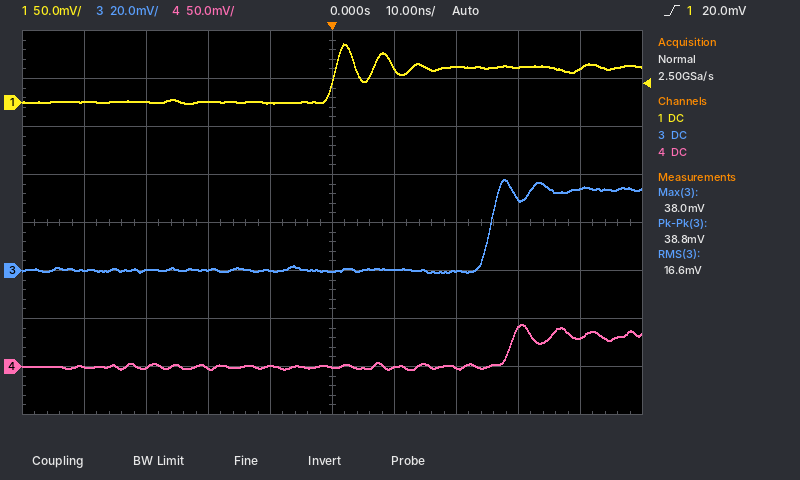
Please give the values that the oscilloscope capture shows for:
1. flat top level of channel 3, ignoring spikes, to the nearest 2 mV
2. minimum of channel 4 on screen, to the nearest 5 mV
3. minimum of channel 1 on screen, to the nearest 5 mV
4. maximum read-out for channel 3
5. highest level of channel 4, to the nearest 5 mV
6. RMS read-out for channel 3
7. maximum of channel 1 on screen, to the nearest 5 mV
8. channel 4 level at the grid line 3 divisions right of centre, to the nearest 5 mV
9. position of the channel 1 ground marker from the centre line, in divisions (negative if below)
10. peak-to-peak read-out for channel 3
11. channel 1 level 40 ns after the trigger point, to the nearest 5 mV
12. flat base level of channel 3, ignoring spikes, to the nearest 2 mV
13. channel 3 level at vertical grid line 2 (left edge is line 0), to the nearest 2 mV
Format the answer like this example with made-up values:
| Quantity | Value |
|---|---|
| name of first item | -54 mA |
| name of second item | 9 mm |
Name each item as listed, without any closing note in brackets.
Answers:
| Quantity | Value |
|---|---|
| flat top level of channel 3, ignoring spikes, to the nearest 2 mV | 34 mV |
| minimum of channel 4 on screen, to the nearest 5 mV | -5 mV |
| minimum of channel 1 on screen, to the nearest 5 mV | 0 mV |
| maximum read-out for channel 3 | 38.0 mV |
| highest level of channel 4, to the nearest 5 mV | 45 mV |
| RMS read-out for channel 3 | 16.6 mV |
| maximum of channel 1 on screen, to the nearest 5 mV | 60 mV |
| channel 4 level at the grid line 3 divisions right of centre, to the nearest 5 mV | 40 mV |
| position of the channel 1 ground marker from the centre line, in divisions | +2.5 div |
| peak-to-peak read-out for channel 3 | 38.8 mV |
| channel 1 level 40 ns after the trigger point, to the nearest 5 mV | 35 mV |
| flat base level of channel 3, ignoring spikes, to the nearest 2 mV | 0 mV |
| channel 3 level at vertical grid line 2 (left edge is line 0), to the nearest 2 mV | 0 mV |
